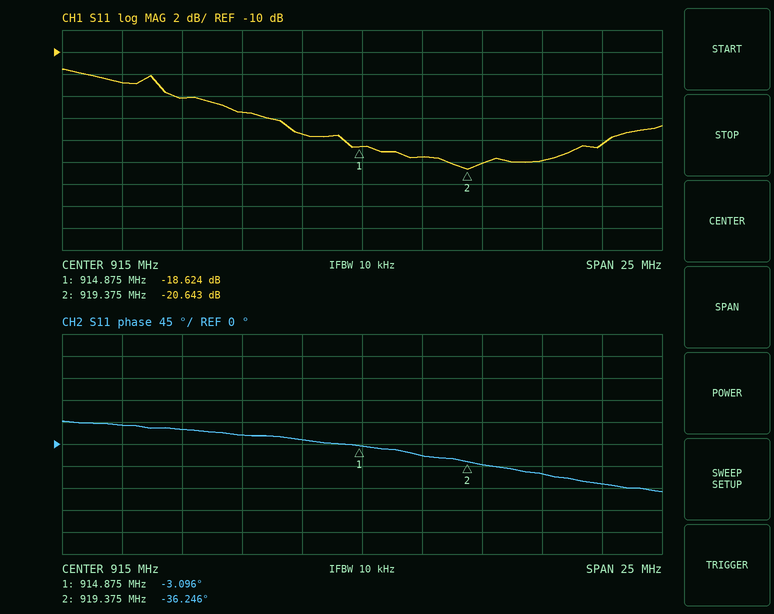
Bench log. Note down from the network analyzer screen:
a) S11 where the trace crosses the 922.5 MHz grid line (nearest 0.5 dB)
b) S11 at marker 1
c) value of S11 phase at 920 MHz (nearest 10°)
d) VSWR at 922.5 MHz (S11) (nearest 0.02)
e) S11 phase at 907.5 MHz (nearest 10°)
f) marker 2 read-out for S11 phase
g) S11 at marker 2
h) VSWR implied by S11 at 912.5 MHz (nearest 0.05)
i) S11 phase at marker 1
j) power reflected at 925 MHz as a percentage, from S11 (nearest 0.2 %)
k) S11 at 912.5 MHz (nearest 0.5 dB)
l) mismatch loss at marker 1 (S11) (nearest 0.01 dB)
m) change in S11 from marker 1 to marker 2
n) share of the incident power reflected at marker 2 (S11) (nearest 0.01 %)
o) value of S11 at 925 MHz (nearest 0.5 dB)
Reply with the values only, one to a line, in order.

-20.0 dB
-18.624 dB
-40°
1.22
30°
-36.246°
-20.643 dB
1.30
-3.096°
1.4 %
-17.5 dB
0.06 dB
-2.019 dB
0.86 %
-18.5 dB
